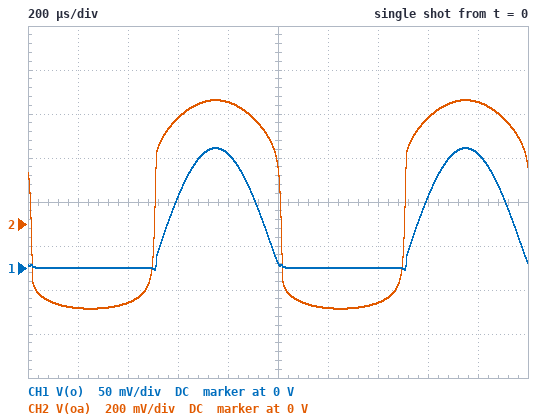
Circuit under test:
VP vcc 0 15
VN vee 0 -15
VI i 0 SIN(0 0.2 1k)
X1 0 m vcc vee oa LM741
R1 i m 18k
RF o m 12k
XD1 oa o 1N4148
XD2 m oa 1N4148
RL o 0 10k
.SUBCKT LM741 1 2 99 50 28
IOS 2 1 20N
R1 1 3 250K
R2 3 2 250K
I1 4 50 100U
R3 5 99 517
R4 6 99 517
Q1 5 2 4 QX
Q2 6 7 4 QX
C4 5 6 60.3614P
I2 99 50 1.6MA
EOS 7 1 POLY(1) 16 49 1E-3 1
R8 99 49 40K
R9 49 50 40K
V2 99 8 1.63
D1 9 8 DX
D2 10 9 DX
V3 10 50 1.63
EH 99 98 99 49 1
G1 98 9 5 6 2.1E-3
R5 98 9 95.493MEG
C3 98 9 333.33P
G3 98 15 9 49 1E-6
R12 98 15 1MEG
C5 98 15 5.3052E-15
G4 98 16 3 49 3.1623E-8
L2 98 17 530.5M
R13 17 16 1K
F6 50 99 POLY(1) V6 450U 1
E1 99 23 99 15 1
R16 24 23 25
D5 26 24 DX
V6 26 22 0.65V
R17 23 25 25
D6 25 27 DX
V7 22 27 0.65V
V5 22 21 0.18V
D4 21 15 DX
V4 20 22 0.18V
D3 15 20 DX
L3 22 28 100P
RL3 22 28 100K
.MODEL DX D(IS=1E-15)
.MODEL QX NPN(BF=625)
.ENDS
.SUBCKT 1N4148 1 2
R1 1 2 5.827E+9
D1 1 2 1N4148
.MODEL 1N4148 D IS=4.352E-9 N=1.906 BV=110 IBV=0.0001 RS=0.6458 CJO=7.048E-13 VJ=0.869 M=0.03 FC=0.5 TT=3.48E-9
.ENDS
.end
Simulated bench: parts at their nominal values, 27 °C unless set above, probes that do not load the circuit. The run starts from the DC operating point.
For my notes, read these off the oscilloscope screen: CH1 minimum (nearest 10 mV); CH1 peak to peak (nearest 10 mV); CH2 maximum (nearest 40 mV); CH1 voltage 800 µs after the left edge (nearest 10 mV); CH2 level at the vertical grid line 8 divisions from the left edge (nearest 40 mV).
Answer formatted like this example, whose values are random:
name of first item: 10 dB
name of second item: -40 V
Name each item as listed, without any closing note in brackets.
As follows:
CH1 minimum: 0 V
CH1 peak to peak: 140 mV
CH2 maximum: 560 mV
CH1 voltage 800 µs after the left edge: 130 mV
CH2 level at the vertical grid line 8 divisions from the left edge: 480 mV
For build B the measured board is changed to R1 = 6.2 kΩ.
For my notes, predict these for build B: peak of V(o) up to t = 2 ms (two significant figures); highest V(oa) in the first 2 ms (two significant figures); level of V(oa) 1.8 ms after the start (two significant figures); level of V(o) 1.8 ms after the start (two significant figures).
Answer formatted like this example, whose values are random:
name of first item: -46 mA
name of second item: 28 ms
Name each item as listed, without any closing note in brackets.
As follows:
peak of V(o) up to t = 2 ms: 390 mV
highest V(oa) in the first 2 ms: 870 mV
level of V(oa) 1.8 ms after the start: 850 mV
level of V(o) 1.8 ms after the start: 370 mV
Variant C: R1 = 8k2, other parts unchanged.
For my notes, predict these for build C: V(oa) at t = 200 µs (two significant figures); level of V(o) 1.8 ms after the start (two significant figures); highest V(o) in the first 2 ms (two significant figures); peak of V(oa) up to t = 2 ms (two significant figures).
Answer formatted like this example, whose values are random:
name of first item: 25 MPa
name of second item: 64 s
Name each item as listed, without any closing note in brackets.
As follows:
V(oa) at t = 200 µs: -420 mV
level of V(o) 1.8 ms after the start: 280 mV
highest V(o) in the first 2 ms: 300 mV
peak of V(oa) up to t = 2 ms: 760 mV
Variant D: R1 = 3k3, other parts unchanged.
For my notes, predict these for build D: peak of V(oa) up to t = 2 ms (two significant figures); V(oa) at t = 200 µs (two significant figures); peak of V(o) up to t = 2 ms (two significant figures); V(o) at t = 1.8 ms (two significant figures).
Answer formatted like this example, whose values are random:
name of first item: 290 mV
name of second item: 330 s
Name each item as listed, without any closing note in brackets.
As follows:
peak of V(oa) up to t = 2 ms: 1.2 V
V(oa) at t = 200 µs: -470 mV
peak of V(o) up to t = 2 ms: 730 mV
V(o) at t = 1.8 ms: 700 mV
